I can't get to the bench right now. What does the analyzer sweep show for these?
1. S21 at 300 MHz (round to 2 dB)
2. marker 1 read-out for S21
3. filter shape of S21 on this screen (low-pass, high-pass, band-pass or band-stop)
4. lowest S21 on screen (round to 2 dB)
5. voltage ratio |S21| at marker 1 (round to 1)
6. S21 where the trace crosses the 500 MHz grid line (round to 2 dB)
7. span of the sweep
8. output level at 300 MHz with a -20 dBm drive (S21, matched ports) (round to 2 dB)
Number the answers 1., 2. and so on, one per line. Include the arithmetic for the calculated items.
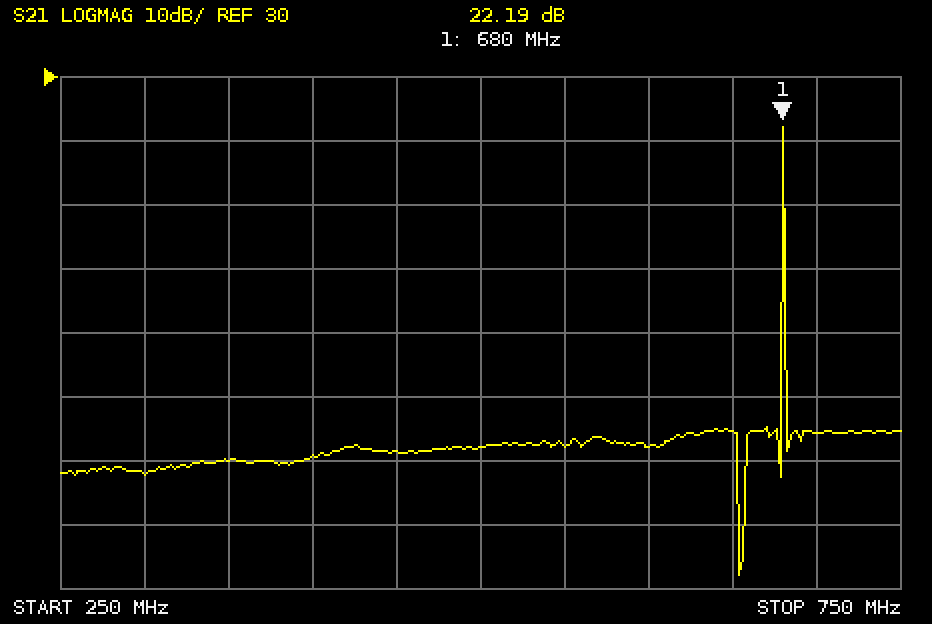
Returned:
1. -32 dB
2. 22.19 dB
3. band-pass
4. -48 dB
5. 10^(22.19/20) ≈ 13
6. -28 dB
7. 500 MHz
8. -20 dBm + (-32 dB) = -52 dBm
